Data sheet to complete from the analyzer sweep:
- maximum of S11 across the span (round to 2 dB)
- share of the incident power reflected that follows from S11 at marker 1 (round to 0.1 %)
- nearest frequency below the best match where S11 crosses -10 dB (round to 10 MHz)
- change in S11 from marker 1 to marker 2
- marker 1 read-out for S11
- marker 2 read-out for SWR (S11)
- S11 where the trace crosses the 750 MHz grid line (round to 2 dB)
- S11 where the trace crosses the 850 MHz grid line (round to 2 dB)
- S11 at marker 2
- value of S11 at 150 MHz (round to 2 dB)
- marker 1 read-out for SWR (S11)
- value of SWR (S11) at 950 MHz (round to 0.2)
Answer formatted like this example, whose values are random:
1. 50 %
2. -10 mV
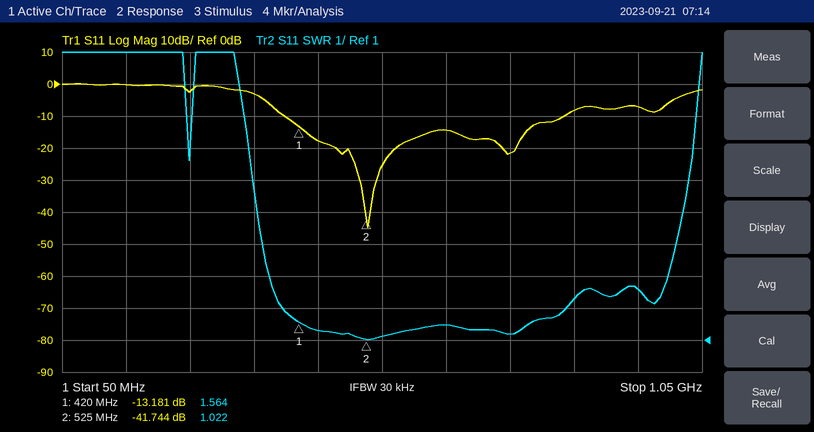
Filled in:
1. 0 dB
2. 4.8 %
3. 400 MHz
4. -28.563 dB
5. -13.181 dB
6. 1.022
7. -22 dB
8. -8 dB
9. -41.744 dB
10. 0 dB
11. 1.564
12. 2.6
